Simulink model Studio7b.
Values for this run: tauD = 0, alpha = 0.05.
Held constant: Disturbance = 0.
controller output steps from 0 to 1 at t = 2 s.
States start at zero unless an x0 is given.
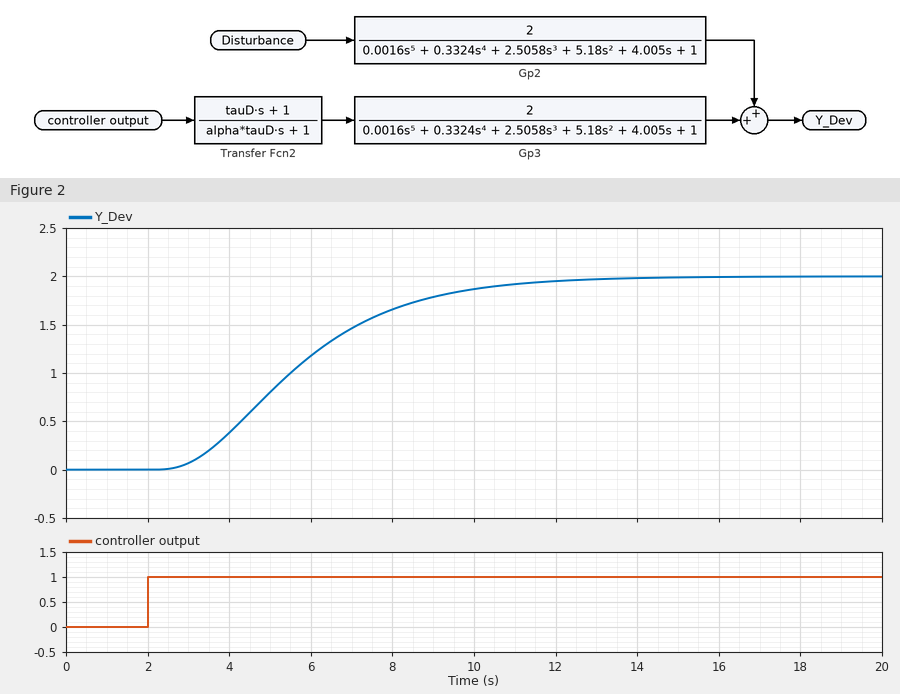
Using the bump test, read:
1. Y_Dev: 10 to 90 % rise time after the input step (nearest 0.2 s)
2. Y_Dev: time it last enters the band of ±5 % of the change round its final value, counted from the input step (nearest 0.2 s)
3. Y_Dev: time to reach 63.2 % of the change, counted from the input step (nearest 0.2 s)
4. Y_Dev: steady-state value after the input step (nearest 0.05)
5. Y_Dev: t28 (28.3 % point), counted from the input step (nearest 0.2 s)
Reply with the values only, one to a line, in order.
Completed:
5.6 s
8.6 s
4.2 s
2.00
2.4 s
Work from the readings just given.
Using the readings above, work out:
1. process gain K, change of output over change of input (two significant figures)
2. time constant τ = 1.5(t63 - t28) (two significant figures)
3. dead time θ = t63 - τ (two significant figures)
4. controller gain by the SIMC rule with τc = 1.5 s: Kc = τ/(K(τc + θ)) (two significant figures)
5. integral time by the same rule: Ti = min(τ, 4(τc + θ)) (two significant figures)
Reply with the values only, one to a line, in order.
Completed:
2.0
2.7 s
1.5 s
0.45
2.7 s
